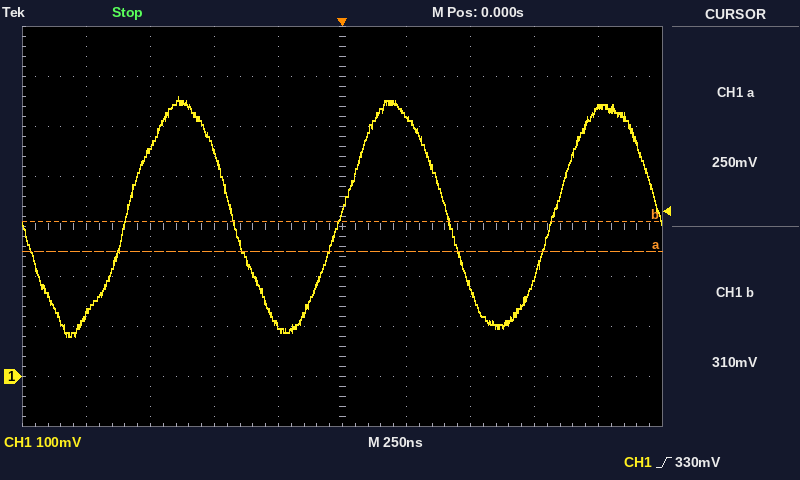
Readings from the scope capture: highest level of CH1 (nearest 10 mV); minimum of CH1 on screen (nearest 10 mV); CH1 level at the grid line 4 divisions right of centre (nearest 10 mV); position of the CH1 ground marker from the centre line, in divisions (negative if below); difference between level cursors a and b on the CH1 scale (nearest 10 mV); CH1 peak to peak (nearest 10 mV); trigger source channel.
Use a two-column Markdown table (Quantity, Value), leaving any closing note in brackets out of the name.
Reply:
| Quantity | Value |
|---|---|
| highest level of CH1 | 560 mV |
| minimum of CH1 on screen | 80 mV |
| CH1 level at the grid line 4 divisions right of centre | 540 mV |
| position of the CH1 ground marker from the centre line, in divisions | -3.0 div |
| difference between level cursors a and b on the CH1 scale | 60 mV |
| CH1 peak to peak | 480 mV |
| trigger source channel | CH1 |
